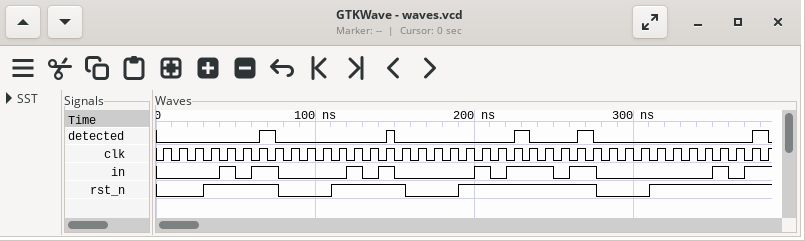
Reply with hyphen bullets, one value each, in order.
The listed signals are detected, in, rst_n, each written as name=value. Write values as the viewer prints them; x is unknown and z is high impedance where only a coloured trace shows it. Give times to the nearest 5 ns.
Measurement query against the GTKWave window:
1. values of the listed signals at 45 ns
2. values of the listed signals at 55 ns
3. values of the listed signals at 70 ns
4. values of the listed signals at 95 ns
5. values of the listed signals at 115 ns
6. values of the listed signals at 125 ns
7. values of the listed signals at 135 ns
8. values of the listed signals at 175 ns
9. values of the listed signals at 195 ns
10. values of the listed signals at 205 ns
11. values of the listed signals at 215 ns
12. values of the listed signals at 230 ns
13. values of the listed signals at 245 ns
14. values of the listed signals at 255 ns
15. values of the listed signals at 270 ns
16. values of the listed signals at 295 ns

- detected=0, in=1, rst_n=1
- detected=0, in=0, rst_n=1
- detected=1, in=1, rst_n=1
- detected=0, in=0, rst_n=0
- detected=0, in=0, rst_n=1
- detected=0, in=1, rst_n=1
- detected=0, in=0, rst_n=1
- detected=0, in=0, rst_n=0
- detected=0, in=0, rst_n=1
- detected=0, in=1, rst_n=1
- detected=0, in=0, rst_n=1
- detected=1, in=1, rst_n=1
- detected=0, in=1, rst_n=1
- detected=0, in=0, rst_n=1
- detected=1, in=1, rst_n=1
- detected=0, in=0, rst_n=0
